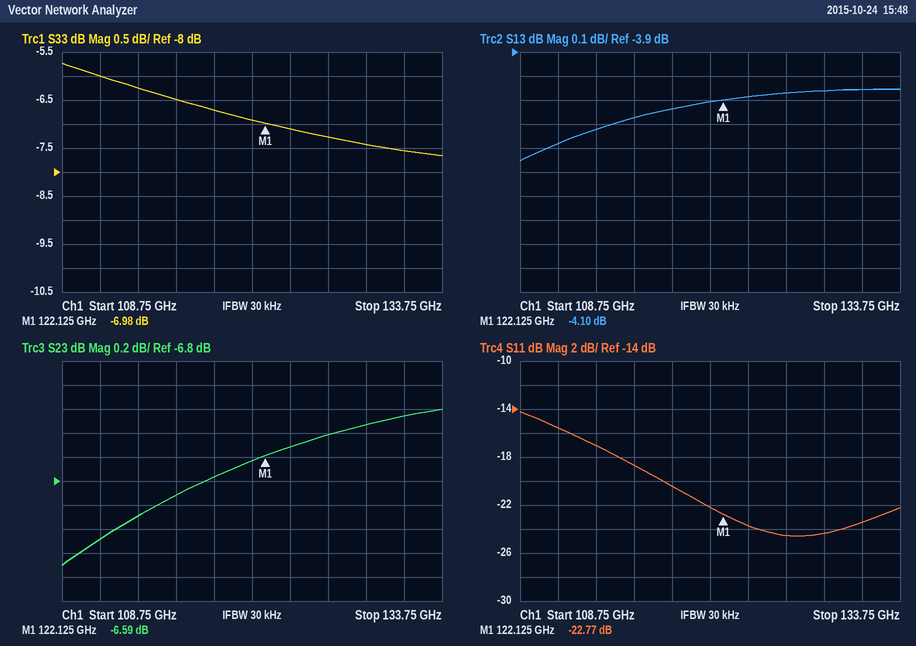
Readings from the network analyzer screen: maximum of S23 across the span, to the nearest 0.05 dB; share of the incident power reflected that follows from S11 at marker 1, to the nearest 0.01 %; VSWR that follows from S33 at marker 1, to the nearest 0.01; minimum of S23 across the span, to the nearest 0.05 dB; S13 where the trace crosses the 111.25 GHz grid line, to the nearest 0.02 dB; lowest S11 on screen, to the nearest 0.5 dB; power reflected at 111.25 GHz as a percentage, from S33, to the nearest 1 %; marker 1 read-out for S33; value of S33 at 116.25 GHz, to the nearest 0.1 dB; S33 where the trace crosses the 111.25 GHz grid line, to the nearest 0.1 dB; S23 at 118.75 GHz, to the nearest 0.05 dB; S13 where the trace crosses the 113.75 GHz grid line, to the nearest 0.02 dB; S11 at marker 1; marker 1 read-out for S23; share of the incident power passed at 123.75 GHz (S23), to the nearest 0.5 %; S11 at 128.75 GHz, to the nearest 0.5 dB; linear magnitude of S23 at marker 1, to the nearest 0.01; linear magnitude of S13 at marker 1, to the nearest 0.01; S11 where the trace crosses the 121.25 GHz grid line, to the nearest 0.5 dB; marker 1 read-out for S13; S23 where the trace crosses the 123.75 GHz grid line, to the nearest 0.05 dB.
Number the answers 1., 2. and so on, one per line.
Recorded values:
1. -6.20 dB
2. 0.53 %
3. 2.62
4. -7.50 dB
5. -4.28 dB
6. -24.5 dB
7. 25 %
8. -6.98 dB
9. -6.5 dB
10. -6.0 dB
11. -6.75 dB
12. -4.22 dB
13. -22.77 dB
14. -6.59 dB
15. 22.5 %
16. -24.5 dB
17. 0.47
18. 0.62
19. -22.0 dB
20. -4.10 dB
21. -6.50 dB
